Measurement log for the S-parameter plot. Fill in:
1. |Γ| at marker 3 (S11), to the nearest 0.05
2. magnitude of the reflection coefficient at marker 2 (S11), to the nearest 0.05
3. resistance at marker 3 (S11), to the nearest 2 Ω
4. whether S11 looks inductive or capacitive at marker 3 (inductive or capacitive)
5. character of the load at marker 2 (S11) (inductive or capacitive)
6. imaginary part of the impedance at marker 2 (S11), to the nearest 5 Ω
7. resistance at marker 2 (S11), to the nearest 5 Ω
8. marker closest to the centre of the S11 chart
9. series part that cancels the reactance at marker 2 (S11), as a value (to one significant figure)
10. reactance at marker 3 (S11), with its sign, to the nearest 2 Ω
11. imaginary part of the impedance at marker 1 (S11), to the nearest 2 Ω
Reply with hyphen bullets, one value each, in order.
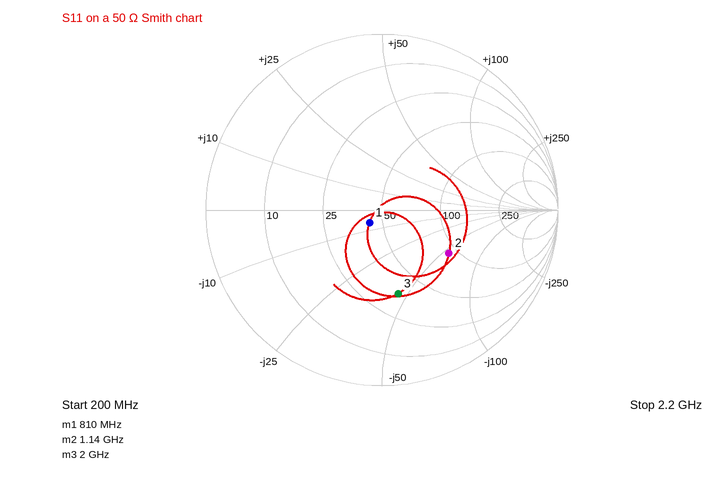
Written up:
- 0.50
- 0.45
- 36 Ω
- capacitive
- capacitive
- -55 Ω
- 90 Ω
- marker 1
- 8 nH
- -46 Ω
- -6 Ω
